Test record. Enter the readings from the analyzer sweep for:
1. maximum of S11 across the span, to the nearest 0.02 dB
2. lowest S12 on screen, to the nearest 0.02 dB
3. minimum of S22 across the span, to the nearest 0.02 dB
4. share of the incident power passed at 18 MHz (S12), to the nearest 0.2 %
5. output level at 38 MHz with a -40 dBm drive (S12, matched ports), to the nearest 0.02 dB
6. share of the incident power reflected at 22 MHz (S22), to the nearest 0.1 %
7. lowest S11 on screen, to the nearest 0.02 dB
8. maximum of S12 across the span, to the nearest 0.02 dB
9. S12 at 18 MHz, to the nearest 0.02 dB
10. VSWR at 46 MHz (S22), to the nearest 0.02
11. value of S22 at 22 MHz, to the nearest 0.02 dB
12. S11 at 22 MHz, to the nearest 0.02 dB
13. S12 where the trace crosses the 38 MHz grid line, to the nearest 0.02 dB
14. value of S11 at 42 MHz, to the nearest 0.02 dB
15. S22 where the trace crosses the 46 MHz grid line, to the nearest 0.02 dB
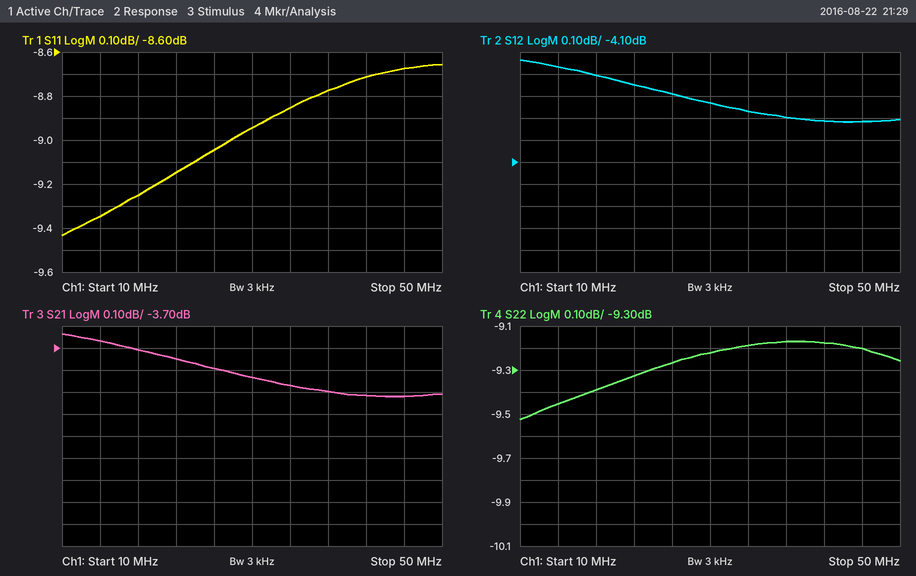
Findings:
-8.66 dB
-3.92 dB
-9.52 dB
42.6 %
-43.90 dBm
11.7 %
-9.44 dB
-3.64 dB
-3.70 dB
2.06
-9.32 dB
-9.14 dB
-3.90 dB
-8.72 dB
-9.20 dB
